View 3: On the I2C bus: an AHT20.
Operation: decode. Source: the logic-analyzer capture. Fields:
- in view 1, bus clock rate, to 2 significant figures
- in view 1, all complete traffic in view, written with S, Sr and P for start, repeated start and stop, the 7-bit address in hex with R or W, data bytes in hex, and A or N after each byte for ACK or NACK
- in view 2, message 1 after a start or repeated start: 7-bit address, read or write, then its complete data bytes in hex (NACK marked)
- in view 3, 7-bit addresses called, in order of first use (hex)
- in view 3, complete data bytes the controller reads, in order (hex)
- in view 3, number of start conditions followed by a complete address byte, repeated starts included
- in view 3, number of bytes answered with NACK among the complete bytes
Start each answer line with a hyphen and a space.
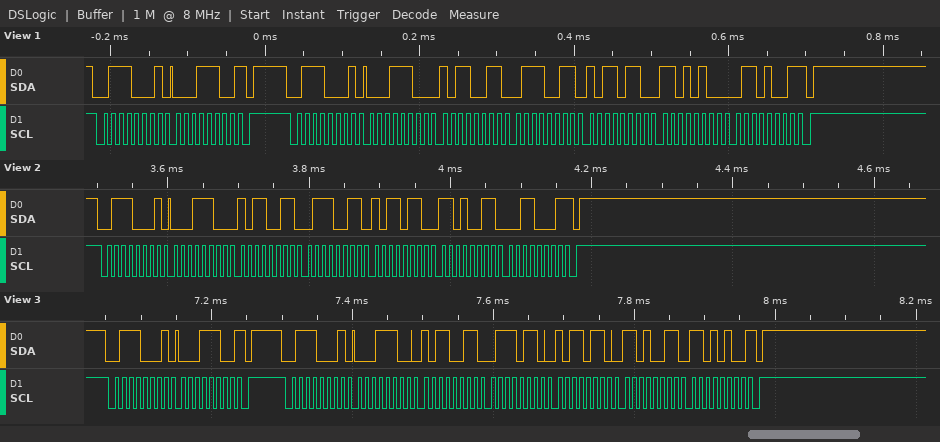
- 100 kHz
- S 38R A 1C N P S 38R A 1C A B3 A 73 A B6 A D4 A 69 N P
- 0x38 read: 1C B3 73 B6 D3 31 NACK
- 0x38
- 1C 1C B3 76 B6 D3 D4
- 2
- 2
